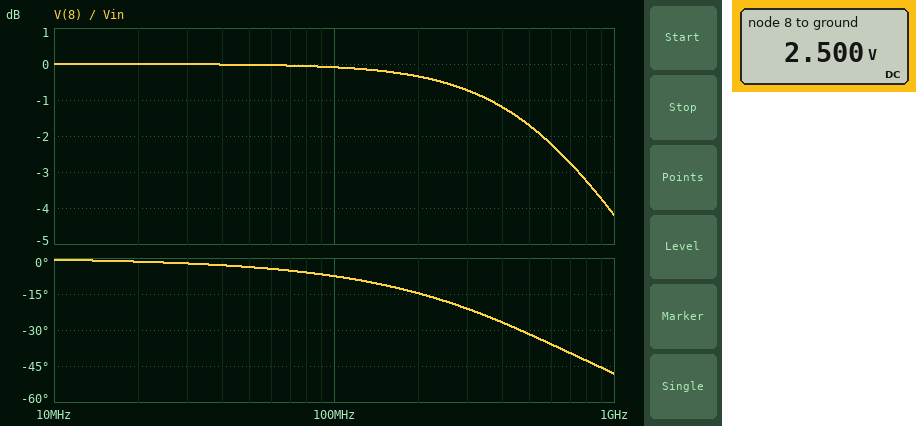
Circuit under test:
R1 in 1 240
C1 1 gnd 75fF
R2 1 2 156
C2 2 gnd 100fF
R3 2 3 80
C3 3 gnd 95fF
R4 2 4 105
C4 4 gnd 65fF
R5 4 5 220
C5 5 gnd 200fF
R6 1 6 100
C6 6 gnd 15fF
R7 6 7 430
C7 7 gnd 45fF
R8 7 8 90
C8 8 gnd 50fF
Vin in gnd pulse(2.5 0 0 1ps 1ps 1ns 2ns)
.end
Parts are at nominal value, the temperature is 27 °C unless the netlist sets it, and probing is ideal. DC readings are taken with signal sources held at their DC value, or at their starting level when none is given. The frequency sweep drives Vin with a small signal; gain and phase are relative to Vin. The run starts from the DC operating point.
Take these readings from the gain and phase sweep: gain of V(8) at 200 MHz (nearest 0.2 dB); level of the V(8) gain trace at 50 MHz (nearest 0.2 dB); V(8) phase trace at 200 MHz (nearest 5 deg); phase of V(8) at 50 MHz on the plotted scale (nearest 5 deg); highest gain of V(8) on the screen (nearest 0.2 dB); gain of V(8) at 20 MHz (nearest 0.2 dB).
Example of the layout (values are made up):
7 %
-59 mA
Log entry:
-0.4 dB
0 dB
-15 deg
-5 deg
0 dB
0 dB
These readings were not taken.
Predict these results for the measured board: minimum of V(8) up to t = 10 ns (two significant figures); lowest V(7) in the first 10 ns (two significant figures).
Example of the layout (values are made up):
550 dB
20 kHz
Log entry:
34 mV
34 mV
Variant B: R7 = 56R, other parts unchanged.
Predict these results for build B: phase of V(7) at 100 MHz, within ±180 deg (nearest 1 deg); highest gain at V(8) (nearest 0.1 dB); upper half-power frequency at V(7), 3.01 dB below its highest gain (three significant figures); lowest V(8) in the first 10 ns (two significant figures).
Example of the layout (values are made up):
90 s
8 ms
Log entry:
-6 deg
0 dB
822 MHz
28 mV
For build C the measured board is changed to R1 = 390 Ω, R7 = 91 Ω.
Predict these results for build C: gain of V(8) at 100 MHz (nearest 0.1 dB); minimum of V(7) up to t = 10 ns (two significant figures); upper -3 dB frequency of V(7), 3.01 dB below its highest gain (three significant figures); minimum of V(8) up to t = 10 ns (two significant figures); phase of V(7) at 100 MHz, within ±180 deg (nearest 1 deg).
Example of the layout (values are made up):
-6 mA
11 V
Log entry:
-0.2 dB
96 mV
523 MHz
97 mV
-10 deg
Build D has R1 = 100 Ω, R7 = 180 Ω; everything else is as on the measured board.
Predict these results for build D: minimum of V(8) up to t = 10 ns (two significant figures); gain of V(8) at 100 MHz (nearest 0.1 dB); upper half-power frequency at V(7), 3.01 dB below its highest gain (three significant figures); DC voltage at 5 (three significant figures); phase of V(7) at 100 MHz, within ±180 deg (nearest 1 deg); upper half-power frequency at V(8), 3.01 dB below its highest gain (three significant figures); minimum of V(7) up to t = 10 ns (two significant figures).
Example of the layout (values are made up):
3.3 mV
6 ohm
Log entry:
2.6 mV
0 dB
1.83 GHz
2.50 V
-3 deg
1.82 GHz
2.5 mV
